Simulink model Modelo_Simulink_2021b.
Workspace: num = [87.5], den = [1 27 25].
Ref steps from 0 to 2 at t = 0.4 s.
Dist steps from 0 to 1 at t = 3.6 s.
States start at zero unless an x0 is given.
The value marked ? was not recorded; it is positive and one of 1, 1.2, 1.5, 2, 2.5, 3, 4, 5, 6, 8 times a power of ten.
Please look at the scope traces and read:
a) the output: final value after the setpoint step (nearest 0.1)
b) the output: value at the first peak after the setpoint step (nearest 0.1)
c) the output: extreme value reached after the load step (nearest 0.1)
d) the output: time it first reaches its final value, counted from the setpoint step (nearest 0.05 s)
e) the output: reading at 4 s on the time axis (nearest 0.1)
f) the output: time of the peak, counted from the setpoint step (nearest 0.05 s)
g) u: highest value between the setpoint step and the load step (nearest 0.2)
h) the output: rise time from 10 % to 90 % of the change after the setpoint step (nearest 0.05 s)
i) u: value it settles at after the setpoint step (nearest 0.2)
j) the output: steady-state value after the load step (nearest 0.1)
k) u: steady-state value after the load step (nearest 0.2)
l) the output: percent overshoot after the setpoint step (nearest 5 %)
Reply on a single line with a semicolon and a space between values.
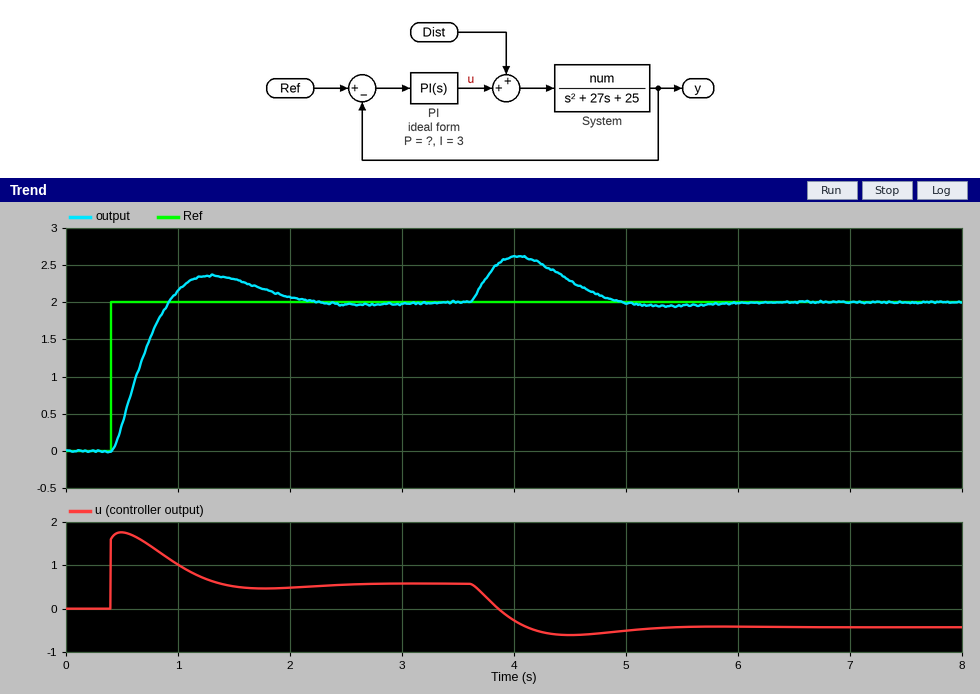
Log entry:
2.0; 2.4; 2.6; 0.50 s; 2.6; 0.90 s; 1.8; 0.35 s; 0.6; 2.0; -0.4; 20 %
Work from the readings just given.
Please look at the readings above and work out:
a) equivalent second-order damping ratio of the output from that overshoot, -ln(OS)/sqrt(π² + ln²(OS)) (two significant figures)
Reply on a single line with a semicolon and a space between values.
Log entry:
0.46
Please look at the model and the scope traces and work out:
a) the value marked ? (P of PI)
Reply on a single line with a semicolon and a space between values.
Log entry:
0.8
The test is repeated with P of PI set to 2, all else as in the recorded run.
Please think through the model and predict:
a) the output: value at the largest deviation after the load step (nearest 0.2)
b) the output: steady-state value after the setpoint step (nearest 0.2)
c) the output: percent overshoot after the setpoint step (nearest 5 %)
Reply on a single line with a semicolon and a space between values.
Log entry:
2.4; 2.0; 15 %
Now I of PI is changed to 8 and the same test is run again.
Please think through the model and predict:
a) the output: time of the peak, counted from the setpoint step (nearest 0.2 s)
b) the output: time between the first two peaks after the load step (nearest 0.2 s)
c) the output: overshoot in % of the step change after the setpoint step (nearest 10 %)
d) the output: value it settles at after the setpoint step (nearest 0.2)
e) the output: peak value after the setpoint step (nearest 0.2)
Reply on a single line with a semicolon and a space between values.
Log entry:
0.6 s; 1.4 s; 40 %; 2.0; 2.8
